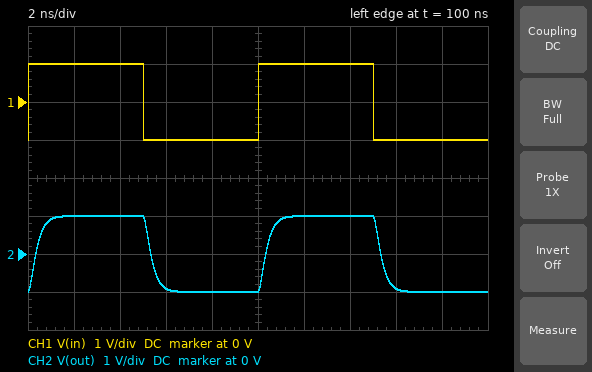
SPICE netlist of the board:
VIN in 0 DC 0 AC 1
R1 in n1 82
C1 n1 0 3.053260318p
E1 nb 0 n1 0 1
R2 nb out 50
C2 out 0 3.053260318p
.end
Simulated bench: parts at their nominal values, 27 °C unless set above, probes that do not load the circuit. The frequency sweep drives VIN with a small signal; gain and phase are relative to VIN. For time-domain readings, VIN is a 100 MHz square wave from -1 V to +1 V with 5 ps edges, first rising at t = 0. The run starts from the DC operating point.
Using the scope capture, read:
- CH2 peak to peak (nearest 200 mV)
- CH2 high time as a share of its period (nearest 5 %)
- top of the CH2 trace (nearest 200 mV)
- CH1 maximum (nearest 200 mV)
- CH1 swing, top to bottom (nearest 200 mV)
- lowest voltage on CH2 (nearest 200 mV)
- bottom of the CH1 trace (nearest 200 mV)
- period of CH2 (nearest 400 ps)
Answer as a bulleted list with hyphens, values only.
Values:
- 2.0 V
- 50 %
- 1.0 V
- 1.0 V
- 2.0 V
- -1.0 V
- -1.0 V
- 10.0 ns
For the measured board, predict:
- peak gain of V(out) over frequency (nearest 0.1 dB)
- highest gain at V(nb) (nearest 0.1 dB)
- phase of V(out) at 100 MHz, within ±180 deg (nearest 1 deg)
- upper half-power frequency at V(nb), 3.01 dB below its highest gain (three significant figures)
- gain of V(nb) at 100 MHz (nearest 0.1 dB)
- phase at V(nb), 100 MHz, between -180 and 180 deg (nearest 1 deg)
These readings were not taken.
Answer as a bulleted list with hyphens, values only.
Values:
- 0 dB
- 0 dB
- -14 deg
- 636 MHz
- -0.1 dB
- -9 deg
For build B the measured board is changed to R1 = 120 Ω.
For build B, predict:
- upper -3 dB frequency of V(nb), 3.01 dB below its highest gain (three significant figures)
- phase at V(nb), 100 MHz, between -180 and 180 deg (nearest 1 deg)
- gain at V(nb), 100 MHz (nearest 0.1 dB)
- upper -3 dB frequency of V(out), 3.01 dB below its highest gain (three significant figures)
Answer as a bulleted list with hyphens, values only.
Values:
- 434 MHz
- -13 deg
- -0.2 dB
- 380 MHz
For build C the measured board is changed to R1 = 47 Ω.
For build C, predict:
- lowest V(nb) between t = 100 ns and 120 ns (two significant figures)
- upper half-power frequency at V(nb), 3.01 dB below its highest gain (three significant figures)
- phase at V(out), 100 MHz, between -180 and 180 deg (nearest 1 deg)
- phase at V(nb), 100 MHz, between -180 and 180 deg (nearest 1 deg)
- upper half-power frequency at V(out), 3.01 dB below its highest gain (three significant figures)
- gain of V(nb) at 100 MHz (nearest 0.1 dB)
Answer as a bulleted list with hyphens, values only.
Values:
- -1.0 V
- 1.11 GHz
- -11 deg
- -5 deg
- 692 MHz
- 0 dB
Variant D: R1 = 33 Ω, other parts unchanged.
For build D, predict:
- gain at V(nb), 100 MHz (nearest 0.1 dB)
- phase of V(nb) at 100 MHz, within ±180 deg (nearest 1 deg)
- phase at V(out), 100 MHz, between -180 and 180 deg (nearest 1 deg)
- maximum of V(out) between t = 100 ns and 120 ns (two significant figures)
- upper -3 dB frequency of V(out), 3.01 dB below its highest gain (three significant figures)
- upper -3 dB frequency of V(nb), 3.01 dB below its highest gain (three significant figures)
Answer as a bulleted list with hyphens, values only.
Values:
- 0 dB
- -4 deg
- -9 deg
- 1.0 V
- 801 MHz
- 1.58 GHz
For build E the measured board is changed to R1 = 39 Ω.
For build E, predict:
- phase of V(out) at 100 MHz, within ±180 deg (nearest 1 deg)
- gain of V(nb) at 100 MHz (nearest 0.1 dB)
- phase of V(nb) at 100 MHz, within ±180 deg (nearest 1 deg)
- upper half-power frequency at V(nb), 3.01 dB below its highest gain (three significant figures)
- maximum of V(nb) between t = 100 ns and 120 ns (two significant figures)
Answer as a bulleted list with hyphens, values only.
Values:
- -10 deg
- 0 dB
- -4 deg
- 1.34 GHz
- 1.0 V
